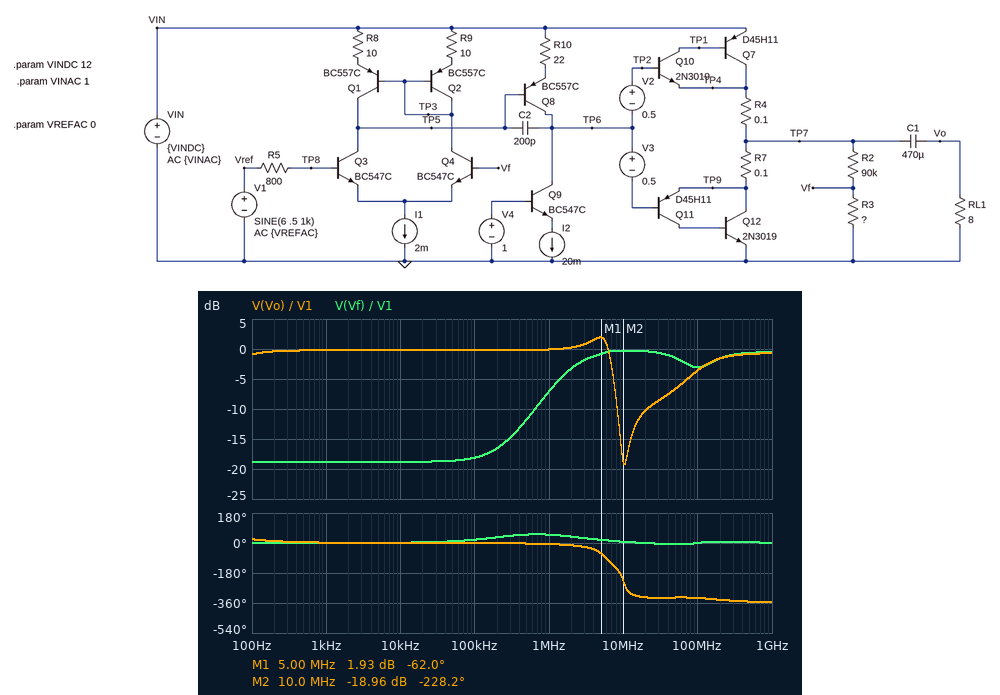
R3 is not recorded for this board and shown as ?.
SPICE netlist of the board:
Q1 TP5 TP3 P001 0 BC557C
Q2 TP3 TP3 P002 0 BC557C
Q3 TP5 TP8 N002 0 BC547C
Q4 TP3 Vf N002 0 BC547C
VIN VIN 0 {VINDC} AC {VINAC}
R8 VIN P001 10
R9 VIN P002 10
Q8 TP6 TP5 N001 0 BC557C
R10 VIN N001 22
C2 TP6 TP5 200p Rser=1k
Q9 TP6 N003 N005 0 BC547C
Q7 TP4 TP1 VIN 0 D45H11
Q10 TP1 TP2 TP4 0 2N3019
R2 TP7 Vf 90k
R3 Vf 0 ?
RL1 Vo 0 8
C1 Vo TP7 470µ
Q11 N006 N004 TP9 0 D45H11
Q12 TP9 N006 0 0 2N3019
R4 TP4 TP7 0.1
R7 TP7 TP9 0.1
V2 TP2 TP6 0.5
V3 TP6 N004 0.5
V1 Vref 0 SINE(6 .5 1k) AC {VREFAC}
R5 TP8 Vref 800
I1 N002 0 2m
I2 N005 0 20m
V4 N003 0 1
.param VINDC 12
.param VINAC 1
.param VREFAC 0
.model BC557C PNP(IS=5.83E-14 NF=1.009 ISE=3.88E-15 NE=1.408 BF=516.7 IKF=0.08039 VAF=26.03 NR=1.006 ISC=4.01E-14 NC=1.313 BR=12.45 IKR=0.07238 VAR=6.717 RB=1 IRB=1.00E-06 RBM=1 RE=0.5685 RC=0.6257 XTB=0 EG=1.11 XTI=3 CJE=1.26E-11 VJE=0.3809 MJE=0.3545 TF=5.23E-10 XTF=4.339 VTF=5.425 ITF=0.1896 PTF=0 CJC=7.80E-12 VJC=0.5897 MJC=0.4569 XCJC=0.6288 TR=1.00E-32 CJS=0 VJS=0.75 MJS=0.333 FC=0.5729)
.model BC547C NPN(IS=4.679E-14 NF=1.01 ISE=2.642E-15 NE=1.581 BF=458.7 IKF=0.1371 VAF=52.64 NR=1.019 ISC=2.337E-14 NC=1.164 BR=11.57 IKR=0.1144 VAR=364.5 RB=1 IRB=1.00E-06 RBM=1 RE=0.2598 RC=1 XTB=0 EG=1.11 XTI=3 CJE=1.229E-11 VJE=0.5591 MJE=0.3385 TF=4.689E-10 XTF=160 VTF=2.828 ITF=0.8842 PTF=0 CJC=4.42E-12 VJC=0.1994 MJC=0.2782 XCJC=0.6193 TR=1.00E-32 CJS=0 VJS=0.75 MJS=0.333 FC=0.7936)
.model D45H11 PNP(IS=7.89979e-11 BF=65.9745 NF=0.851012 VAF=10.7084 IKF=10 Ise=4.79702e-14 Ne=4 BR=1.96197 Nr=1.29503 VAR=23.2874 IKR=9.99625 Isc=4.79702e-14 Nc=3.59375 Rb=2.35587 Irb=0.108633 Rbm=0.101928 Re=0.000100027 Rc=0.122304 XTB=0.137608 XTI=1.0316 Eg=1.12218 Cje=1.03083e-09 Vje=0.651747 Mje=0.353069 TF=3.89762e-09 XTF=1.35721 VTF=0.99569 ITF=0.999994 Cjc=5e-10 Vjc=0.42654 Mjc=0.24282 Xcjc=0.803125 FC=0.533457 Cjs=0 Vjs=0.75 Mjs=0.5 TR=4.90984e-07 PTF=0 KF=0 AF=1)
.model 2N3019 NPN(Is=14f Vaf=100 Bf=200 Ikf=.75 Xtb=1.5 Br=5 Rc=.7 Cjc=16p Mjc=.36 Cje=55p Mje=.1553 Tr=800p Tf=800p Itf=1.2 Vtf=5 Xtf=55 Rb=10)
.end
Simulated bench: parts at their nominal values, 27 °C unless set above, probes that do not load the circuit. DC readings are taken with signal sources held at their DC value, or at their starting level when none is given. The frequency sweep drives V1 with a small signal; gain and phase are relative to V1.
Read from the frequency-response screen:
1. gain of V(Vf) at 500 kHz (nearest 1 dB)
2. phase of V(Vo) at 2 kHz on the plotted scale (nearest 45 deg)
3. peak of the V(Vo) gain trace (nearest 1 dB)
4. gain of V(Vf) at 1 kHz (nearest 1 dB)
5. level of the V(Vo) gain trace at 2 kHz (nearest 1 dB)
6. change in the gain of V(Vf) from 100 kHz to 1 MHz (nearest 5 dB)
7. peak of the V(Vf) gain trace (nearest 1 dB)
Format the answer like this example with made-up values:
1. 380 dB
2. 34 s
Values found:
1. -12 dB
2. 0 deg
3. 2 dB
4. -19 dB
5. 0 dB
6. 10 dB
7. 0 dB
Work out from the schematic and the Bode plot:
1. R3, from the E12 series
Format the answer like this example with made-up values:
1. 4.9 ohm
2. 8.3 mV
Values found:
1. 12 kΩ
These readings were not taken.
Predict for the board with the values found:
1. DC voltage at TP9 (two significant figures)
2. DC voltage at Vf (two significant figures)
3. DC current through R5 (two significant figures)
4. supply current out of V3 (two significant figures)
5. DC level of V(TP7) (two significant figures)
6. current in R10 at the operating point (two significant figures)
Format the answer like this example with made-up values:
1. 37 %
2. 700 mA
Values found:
1. 11 V
2. 1.3 V
3. 4.1 µA
4. 3.5 µA
5. 11 V
6. 22 mA
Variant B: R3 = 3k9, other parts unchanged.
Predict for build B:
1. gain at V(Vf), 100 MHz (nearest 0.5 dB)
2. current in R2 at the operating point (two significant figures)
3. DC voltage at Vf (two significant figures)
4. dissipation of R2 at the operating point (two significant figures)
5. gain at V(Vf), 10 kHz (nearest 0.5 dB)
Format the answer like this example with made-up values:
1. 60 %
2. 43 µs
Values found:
1. -3.5 dB
2. 120 µA
3. 470 mV
4. 1.3 mW
5. -28.0 dB
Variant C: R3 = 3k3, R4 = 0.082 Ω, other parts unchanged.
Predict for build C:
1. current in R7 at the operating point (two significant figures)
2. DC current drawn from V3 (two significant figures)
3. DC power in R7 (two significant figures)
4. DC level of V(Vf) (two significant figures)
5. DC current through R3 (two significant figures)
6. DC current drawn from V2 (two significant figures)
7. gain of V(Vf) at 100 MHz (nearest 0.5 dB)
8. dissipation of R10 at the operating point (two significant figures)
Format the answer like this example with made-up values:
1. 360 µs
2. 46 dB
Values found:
1. 92 mA
2. 3.6 µA
3. 840 µW
4. 400 mV
5. 120 µA
6. 7.0 µA
7. -3.5 dB
8. 11 mW
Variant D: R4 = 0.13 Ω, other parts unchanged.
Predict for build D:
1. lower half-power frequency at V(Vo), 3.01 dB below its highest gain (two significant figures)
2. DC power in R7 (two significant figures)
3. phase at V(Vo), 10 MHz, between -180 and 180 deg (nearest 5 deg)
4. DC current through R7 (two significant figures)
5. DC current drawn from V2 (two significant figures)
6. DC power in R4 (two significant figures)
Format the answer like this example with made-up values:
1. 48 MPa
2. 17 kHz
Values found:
1. 89 Hz
2. 740 µW
3. 125 deg
4. 86 mA
5. 6.6 µA
6. 970 µW
